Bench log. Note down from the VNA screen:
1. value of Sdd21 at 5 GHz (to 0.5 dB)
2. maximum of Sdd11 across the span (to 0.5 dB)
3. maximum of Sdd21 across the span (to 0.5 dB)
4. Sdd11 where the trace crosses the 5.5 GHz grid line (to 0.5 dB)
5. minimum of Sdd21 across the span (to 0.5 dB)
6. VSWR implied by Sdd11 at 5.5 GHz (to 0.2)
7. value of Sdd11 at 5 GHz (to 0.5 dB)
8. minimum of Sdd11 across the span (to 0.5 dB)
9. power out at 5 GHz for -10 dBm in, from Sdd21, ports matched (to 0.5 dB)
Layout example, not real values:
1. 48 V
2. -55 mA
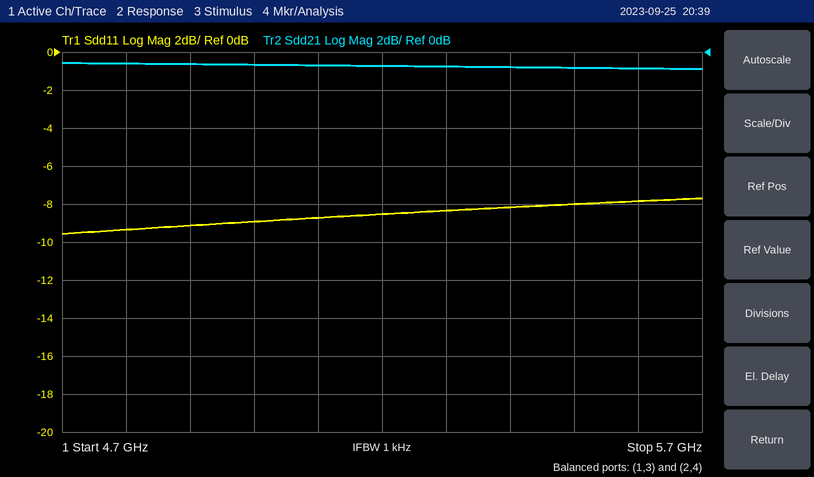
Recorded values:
1. -0.5 dB
2. -7.5 dB
3. -0.5 dB
4. -8.0 dB
5. -1.0 dB
6. 2.4
7. -9.0 dB
8. -9.5 dB
9. -10.5 dBm
